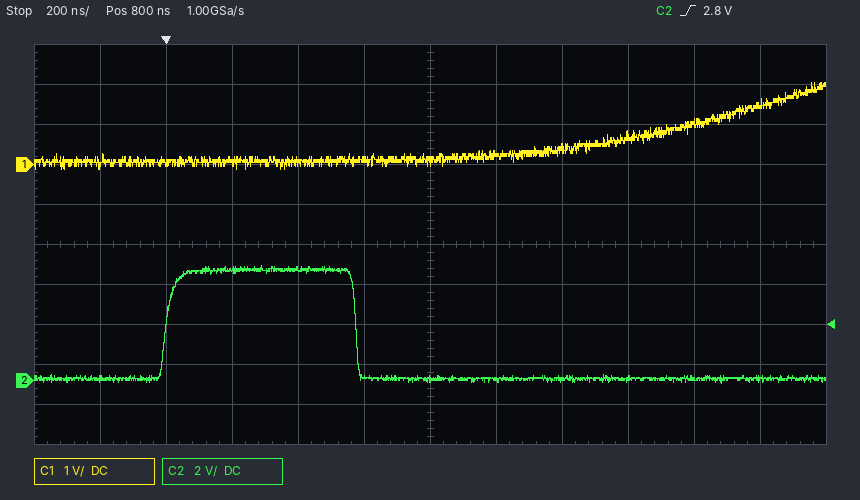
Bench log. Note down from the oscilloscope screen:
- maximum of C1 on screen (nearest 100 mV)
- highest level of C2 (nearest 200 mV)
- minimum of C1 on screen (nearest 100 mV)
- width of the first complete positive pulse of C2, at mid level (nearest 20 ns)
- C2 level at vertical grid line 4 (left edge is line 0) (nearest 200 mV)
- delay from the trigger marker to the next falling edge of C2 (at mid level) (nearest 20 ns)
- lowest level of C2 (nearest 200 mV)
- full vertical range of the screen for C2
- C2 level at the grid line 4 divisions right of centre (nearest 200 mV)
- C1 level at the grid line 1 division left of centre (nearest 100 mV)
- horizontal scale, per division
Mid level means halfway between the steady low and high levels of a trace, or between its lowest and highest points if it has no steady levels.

2.0 V
5.8 V
-100 mV
580 ns
5.6 V
580 ns
-200 mV
20 V
200 mV
100 mV
200 ns
